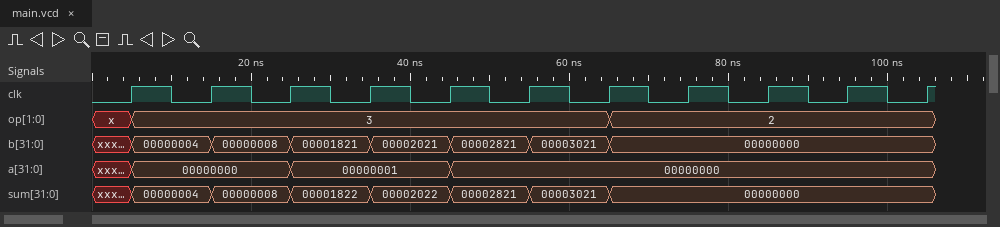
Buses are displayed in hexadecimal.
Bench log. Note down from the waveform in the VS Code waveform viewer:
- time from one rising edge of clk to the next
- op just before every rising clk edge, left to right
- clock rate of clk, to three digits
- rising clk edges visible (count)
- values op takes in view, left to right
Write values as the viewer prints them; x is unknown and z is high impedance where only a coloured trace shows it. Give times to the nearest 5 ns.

10 ns
x, 3, 3, 3, 3, 3, 3, 2, 2, 2, 2
100 MHz
11
x, 3, 2
